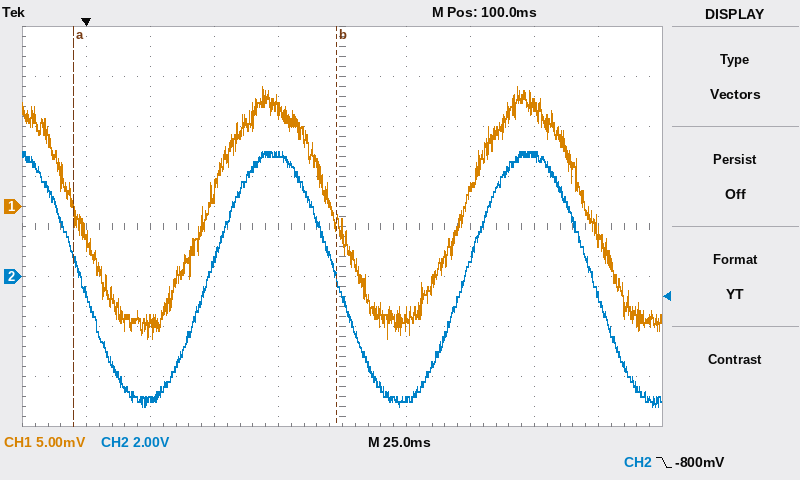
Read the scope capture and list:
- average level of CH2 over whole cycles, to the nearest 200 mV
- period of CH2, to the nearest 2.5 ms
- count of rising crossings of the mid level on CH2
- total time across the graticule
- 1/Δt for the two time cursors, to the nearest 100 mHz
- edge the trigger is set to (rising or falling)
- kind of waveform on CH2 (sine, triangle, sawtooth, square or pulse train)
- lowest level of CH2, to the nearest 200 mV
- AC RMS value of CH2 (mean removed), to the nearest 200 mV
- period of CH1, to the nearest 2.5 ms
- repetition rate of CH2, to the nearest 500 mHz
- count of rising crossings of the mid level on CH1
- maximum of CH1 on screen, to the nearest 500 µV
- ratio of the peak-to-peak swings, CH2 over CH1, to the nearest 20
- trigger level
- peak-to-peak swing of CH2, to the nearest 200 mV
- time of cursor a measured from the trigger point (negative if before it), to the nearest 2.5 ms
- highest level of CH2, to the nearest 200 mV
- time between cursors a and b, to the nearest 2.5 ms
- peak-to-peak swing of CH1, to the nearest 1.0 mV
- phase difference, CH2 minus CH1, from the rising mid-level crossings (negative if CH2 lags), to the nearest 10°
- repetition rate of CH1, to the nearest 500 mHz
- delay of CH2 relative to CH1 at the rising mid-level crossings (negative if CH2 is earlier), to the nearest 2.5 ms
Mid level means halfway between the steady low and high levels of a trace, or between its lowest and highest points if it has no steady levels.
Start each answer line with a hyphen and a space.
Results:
- 0.0 V
- 100.0 ms
- 2
- 250 ms
- 9.8 Hz
- falling
- sine
- -5.2 V
- 3.6 V
- 100.0 ms
- 10.0 Hz
- 2
- 12.0 mV
- 400
- -800 mV
- 10.2 V
- -5.0 ms
- 5.0 V
- 102.5 ms
- 25.0 mV
- 0°
- 10.0 Hz
- 0.0 ms
